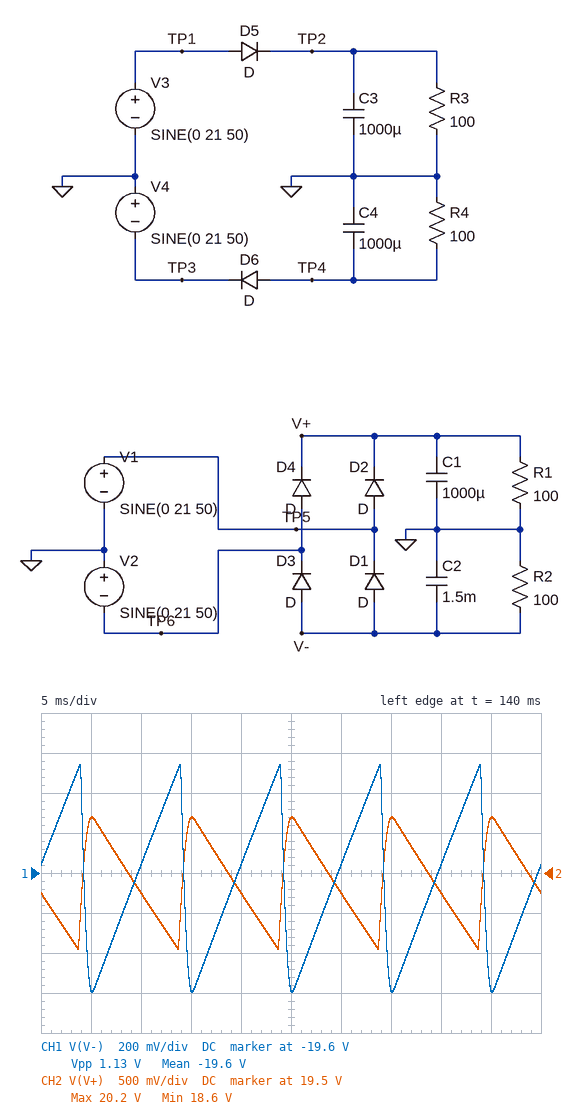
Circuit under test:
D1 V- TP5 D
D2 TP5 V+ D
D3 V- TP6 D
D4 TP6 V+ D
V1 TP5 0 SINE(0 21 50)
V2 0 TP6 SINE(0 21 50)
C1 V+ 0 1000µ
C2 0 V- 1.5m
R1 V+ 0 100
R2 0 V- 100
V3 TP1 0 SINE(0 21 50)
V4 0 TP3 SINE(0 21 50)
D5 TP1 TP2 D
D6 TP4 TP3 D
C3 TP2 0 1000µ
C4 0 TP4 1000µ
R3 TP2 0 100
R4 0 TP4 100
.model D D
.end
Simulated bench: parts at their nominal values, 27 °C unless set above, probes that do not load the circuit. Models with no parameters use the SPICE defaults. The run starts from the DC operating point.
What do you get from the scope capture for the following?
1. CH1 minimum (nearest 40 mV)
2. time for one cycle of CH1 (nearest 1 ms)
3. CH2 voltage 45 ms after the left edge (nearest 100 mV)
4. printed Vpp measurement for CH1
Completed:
-20.20 V
10 ms
20.2 V
1.13 V
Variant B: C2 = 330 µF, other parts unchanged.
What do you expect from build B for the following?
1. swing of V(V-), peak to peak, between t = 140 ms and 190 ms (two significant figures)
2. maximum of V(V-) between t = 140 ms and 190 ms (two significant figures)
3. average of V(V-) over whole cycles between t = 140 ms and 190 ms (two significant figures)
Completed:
4.2 V
-16 V
-18 V
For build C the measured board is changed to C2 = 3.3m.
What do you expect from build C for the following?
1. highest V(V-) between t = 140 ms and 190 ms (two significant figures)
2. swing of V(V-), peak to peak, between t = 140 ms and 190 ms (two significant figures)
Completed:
-20 V
540 mV
